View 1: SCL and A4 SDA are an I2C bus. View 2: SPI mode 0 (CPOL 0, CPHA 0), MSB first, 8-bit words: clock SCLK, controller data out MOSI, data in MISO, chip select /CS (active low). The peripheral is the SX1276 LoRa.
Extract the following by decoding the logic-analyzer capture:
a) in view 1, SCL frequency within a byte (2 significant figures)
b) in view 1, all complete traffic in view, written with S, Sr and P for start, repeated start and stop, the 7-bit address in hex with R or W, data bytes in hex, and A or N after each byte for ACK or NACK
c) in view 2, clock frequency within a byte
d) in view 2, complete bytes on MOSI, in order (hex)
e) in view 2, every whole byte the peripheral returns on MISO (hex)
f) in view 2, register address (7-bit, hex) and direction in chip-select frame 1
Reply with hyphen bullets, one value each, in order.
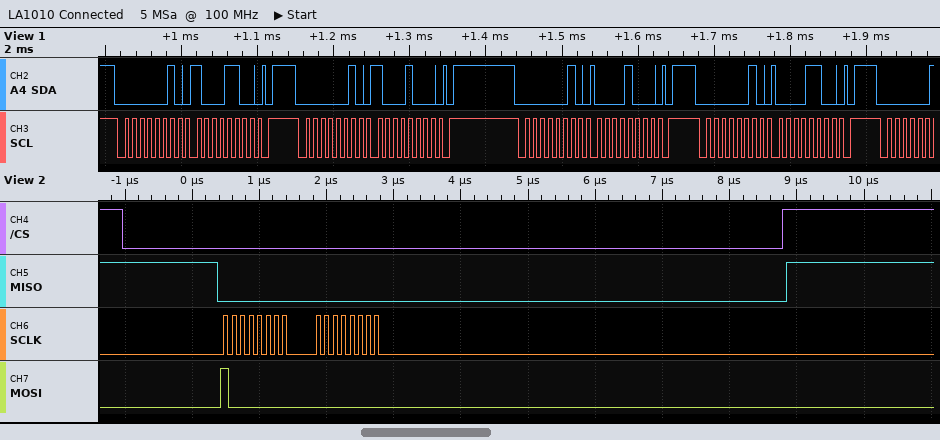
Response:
- 100 kHz
- S 01W A 8C A P S 01W A 88 A P S 01W A 08 A P S 01W A 0C A P
- 8 MHz
- 0x80 0x00
- 0x00 0x00
- 0x00 write
